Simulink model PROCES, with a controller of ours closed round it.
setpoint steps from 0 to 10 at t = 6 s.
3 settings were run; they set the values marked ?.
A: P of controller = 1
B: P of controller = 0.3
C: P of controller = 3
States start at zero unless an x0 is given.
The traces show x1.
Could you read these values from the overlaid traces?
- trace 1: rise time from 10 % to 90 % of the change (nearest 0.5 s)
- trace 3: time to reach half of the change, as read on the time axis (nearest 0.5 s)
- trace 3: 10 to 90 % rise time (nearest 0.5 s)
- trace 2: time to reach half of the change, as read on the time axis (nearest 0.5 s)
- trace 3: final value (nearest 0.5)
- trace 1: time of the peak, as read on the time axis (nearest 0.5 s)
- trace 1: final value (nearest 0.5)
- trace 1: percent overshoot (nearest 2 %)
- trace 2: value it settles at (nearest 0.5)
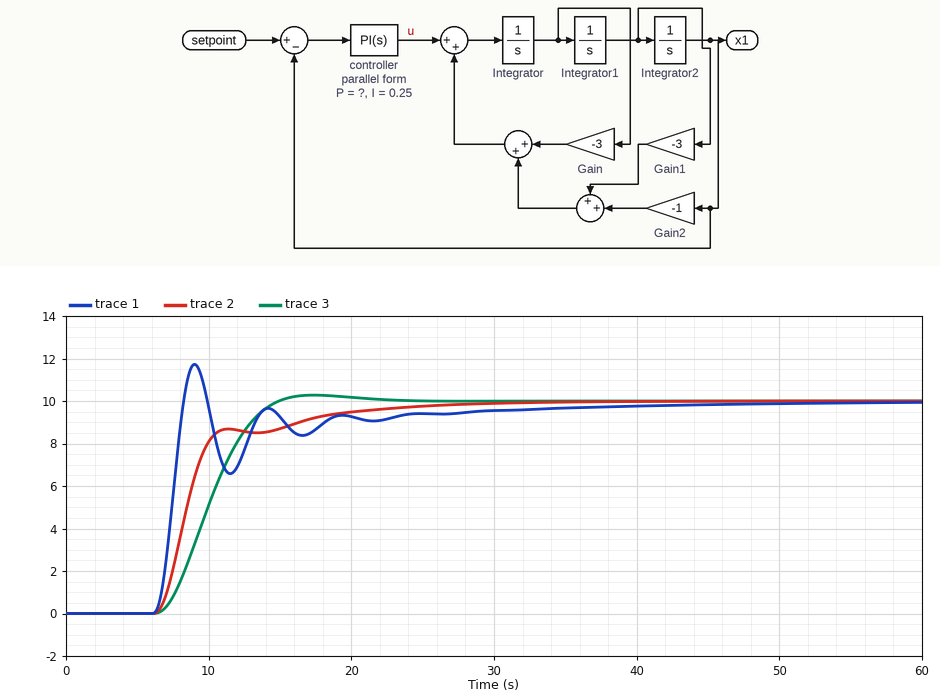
1.5 s
10.0 s
5.5 s
8.5 s
10.0
9.0 s
10.0
18 %
10.0
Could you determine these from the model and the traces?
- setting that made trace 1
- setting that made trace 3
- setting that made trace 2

C
B
A
